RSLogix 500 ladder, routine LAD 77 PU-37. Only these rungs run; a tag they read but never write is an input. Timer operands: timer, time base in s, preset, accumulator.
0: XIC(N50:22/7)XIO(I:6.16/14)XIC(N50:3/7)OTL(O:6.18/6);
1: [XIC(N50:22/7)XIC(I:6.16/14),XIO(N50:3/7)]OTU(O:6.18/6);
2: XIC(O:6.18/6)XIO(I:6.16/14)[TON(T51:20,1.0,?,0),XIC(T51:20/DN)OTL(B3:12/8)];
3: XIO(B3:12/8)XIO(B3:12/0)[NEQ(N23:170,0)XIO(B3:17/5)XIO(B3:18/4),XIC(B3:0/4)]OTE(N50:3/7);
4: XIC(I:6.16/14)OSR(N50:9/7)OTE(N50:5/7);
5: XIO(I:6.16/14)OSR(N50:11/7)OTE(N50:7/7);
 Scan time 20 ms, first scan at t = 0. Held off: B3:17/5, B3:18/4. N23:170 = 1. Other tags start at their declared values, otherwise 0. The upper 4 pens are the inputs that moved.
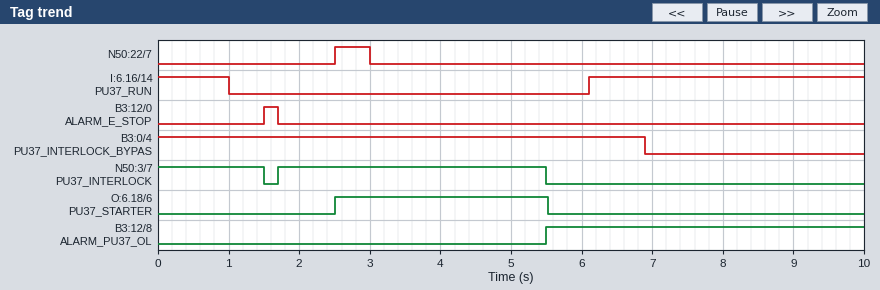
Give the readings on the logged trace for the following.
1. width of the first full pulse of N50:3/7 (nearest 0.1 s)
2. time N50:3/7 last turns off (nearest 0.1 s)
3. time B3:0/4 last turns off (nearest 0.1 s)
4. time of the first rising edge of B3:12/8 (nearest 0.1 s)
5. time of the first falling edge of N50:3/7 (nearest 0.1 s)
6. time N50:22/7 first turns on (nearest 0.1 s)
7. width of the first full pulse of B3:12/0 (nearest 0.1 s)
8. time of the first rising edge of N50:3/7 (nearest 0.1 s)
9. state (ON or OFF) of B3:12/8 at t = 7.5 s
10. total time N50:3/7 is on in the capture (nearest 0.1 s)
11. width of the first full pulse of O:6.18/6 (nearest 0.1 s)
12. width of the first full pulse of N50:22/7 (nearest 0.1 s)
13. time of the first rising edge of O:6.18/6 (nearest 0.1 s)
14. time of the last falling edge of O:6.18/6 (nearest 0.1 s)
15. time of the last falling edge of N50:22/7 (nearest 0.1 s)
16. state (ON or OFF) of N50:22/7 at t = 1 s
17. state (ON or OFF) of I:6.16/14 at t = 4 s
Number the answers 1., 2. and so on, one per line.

1. 3.8 s
2. 5.5 s
3. 6.9 s
4. 5.5 s
5. 1.5 s
6. 2.5 s
7. 0.2 s
8. 1.7 s
9. ON
10. 5.3 s
11. 3.0 s
12. 0.5 s
13. 2.5 s
14. 5.5 s
15. 3.0 s
16. OFF
17. OFF
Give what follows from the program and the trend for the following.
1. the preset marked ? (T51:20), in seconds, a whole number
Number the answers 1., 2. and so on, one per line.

1. 3 s
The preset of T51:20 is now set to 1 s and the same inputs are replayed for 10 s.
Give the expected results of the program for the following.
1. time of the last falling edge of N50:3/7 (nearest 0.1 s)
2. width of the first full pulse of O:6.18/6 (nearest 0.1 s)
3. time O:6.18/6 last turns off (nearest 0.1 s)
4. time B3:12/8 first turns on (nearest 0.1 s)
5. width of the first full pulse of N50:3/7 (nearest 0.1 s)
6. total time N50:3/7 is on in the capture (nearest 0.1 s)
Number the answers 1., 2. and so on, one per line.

1. 3.5 s
2. 1.0 s
3. 3.5 s
4. 3.5 s
5. 1.8 s
6. 3.3 s
